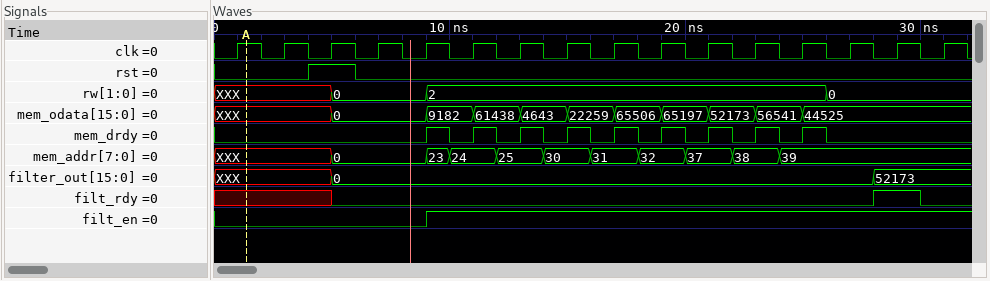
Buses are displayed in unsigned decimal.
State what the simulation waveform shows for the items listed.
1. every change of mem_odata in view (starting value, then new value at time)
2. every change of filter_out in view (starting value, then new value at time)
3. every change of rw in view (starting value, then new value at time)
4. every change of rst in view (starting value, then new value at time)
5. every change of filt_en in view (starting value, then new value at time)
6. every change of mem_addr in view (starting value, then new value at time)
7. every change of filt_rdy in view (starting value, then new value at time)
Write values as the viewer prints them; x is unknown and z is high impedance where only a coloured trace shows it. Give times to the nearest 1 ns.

XXX, 0 at 5 ns, 9182 at 9 ns, 61438 at 11 ns, 4643 at 13 ns, 22259 at 15 ns, 65506 at 17 ns, 65197 at 19 ns, 52173 at 21 ns, 56541 at 23 ns, 44525 at 25 ns
XXX, 0 at 5 ns, 52173 at 28 ns
XXX, 0 at 5 ns, 2 at 9 ns, 0 at 26 ns
0, 1 at 4 ns, 0 at 6 ns
0, 1 at 9 ns
XXX, 0 at 5 ns, 23 at 9 ns, 24 at 10 ns, 25 at 12 ns, 30 at 14 ns, 31 at 16 ns, 32 at 18 ns, 37 at 20 ns, 38 at 22 ns, 39 at 24 ns
x, 0 at 5 ns, 1 at 28 ns, 0 at 30 ns
